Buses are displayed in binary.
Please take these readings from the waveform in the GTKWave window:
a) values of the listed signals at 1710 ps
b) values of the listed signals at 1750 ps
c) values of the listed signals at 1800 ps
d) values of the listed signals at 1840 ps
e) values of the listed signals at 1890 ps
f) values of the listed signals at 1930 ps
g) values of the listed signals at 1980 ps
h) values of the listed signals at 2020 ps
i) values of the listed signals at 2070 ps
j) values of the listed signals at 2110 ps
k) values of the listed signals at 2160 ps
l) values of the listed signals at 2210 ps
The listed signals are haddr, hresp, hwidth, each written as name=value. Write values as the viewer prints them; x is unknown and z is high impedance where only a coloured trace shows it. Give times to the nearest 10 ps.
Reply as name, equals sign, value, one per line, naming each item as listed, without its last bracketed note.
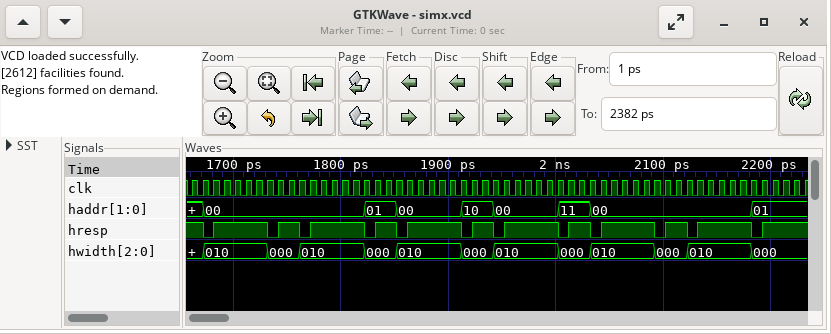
values of the listed signals at 1710 ps = haddr=00, hresp=1, hwidth=010
values of the listed signals at 1750 ps = haddr=00, hresp=1, hwidth=000
values of the listed signals at 1800 ps = haddr=00, hresp=1, hwidth=010
values of the listed signals at 1840 ps = haddr=01, hresp=1, hwidth=000
values of the listed signals at 1890 ps = haddr=00, hresp=1, hwidth=010
values of the listed signals at 1930 ps = haddr=10, hresp=1, hwidth=000
values of the listed signals at 1980 ps = haddr=00, hresp=1, hwidth=010
values of the listed signals at 2020 ps = haddr=11, hresp=1, hwidth=000
values of the listed signals at 2070 ps = haddr=00, hresp=1, hwidth=010
values of the listed signals at 2110 ps = haddr=00, hresp=1, hwidth=000
values of the listed signals at 2160 ps = haddr=00, hresp=1, hwidth=010
values of the listed signals at 2210 ps = haddr=01, hresp=1, hwidth=000
